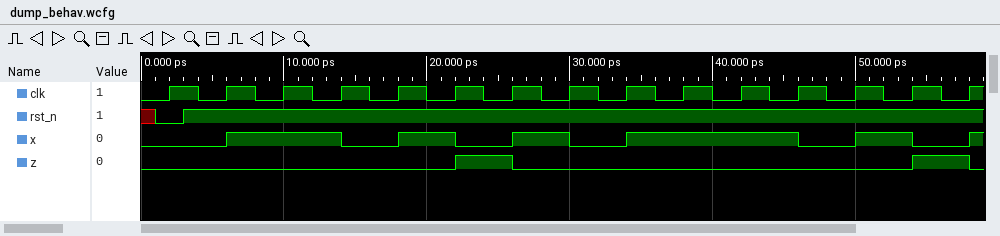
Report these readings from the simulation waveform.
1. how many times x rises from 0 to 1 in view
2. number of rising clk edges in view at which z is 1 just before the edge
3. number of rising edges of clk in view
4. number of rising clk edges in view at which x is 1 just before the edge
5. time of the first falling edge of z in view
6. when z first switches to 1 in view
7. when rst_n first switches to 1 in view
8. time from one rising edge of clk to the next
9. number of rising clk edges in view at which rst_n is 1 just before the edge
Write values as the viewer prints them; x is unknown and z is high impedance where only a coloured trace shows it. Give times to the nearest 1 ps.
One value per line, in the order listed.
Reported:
6
2
15
8
26 ps
22 ps
3 ps
4 ps
14
